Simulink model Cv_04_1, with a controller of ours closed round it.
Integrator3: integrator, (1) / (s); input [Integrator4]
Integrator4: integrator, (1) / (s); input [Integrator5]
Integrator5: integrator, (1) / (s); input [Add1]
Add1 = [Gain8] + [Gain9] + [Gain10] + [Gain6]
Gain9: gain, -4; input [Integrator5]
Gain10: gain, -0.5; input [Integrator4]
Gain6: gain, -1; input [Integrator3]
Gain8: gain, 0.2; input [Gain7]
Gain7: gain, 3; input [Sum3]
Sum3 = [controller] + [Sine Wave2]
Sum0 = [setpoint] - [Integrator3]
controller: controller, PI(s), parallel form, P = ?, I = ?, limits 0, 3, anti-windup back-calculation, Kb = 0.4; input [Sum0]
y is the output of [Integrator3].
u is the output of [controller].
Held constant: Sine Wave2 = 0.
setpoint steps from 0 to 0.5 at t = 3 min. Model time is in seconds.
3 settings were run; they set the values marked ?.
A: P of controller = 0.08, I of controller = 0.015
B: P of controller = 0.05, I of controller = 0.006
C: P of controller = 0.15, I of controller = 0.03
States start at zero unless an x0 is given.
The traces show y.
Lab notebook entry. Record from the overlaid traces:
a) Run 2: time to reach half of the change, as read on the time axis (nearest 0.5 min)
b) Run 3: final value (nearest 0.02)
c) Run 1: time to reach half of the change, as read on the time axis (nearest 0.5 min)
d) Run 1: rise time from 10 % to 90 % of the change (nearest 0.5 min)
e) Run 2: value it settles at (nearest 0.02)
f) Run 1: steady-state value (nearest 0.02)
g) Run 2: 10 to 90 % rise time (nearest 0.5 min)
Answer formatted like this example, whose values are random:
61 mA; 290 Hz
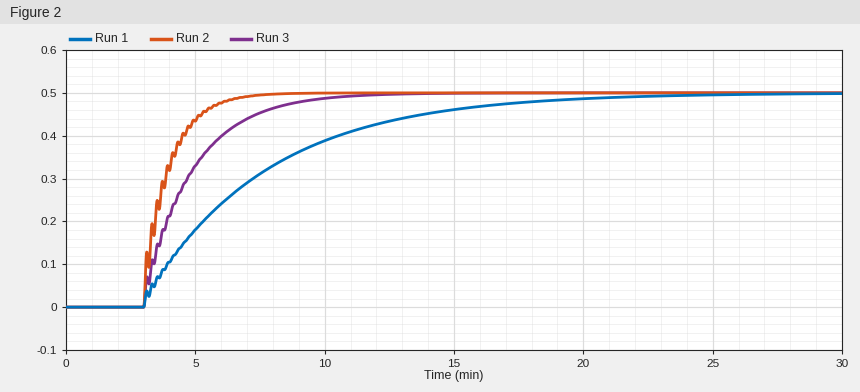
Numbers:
3.5 min; 0.50; 6.0 min; 10.5 min; 0.50; 0.50; 2.0 min
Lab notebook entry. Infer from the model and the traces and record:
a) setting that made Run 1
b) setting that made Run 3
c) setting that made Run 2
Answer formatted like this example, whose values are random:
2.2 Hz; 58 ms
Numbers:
B; A; C
